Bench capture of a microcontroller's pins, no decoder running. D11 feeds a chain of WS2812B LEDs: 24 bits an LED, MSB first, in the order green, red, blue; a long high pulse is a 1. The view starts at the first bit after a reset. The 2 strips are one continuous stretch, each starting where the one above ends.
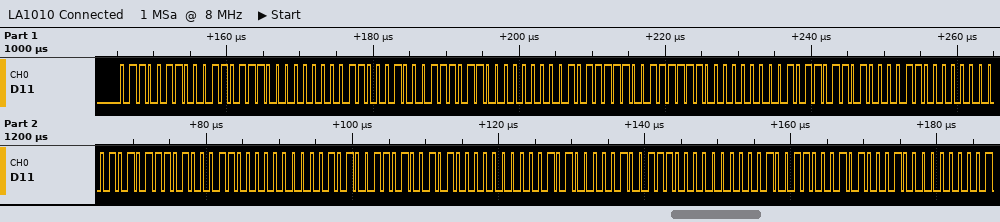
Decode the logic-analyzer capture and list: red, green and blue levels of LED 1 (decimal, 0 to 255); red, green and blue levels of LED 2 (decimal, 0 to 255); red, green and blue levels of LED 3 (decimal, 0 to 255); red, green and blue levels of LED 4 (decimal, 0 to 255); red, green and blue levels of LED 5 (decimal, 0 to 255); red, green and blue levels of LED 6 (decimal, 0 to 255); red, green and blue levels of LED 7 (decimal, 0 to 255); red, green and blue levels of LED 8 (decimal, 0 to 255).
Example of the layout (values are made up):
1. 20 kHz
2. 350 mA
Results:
1. 55, 102, 0
2. 59, 98, 0
3. 63, 95, 0
4. 67, 91, 0
5. 70, 87, 0
6. 74, 83, 0
7. 78, 80, 0
8. 81, 76, 0
